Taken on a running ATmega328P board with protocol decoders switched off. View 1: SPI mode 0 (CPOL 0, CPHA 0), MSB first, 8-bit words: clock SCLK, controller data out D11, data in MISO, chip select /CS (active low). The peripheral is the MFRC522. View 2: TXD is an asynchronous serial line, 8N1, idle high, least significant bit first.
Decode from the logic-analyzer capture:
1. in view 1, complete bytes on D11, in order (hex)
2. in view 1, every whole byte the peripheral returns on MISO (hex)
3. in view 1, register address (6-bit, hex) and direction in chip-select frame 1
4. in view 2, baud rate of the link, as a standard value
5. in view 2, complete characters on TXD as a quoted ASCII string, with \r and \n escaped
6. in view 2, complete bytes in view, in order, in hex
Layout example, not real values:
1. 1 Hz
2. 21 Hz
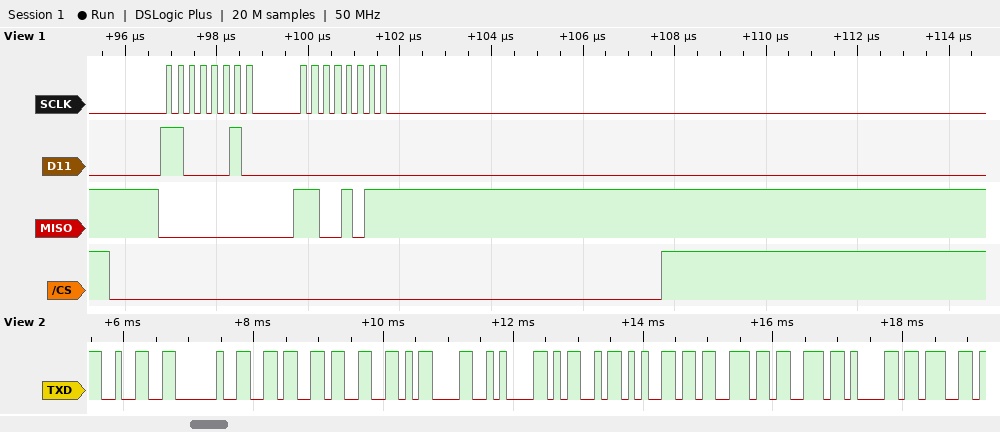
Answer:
1. C2 00
2. 00 CB
3. 0x21 read
4. 9600 baud
5. "2 63\r\nMessag"
6. 32 20 36 33 0D 0A 4D 65 73 73 61 67
